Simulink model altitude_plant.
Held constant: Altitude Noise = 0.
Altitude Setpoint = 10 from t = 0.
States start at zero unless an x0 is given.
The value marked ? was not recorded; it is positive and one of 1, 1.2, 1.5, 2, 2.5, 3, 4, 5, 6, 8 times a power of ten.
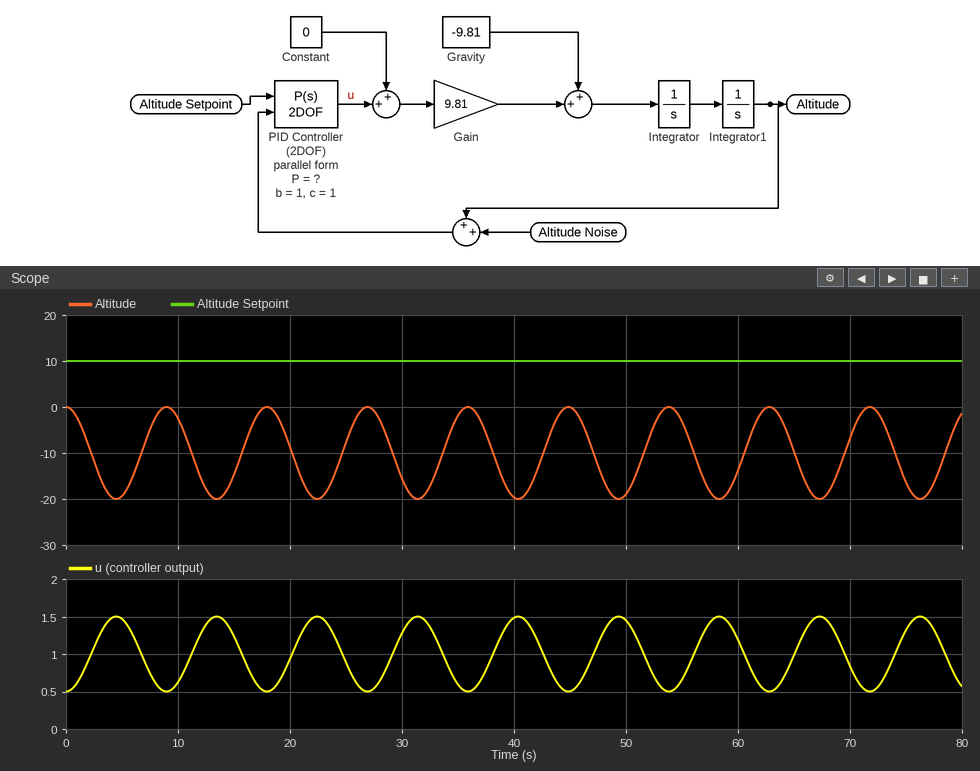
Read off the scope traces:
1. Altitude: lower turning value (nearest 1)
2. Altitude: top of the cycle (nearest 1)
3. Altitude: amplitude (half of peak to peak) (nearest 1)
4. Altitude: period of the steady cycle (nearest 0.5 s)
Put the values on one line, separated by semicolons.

-20; 0; 10; 9.0 s
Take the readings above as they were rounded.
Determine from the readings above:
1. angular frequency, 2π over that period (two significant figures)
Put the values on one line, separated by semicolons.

0.70 rad/s
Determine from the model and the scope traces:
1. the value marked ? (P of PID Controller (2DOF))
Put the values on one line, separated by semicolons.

0.05
